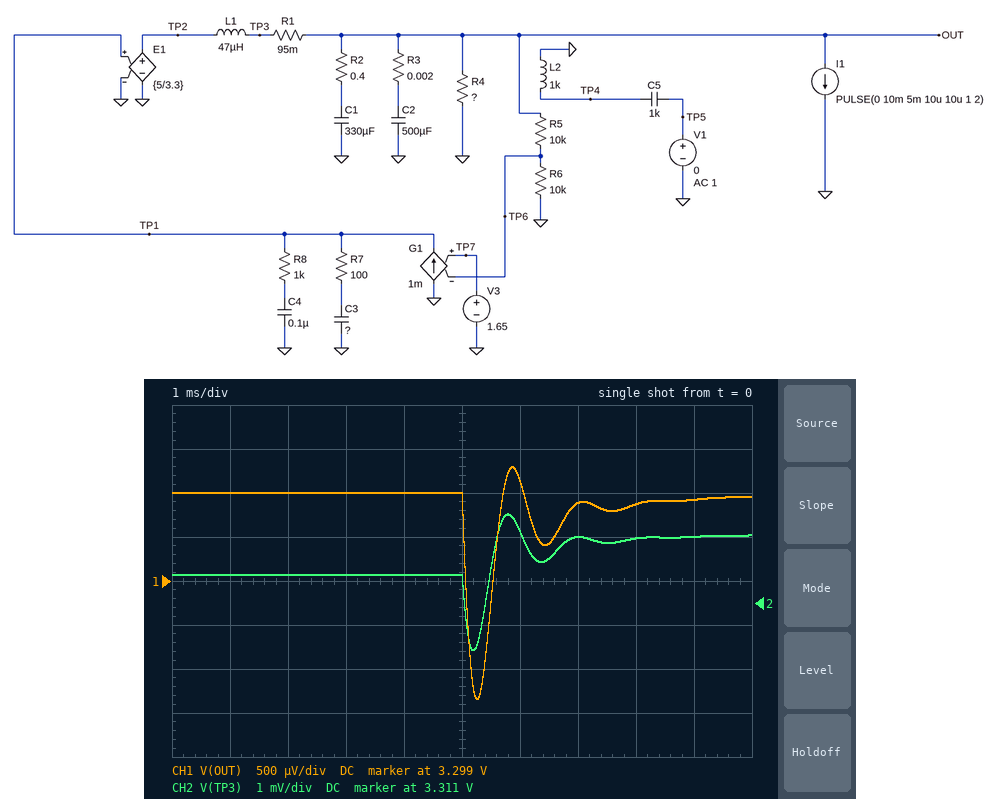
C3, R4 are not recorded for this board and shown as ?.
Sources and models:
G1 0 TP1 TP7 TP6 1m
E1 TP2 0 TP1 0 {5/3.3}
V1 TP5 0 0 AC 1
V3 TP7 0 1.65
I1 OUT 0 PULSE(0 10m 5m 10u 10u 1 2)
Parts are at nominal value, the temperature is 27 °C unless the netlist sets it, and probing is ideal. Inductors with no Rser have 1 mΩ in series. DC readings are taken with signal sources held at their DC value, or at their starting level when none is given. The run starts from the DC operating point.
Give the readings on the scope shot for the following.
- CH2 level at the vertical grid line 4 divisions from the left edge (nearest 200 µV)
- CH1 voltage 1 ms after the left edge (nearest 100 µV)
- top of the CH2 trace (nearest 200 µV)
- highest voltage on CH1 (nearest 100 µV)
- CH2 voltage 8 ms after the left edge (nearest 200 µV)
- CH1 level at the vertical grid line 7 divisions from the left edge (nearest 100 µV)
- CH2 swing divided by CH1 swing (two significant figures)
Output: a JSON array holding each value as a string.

["3.3116 V", "3.3000 V", "3.3130 V", "3.3003 V", "3.3124 V", "3.2999 V", "1.2"]
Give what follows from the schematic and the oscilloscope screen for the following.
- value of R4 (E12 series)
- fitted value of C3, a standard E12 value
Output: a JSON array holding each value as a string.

["27 Ω", "1.2 µF"]
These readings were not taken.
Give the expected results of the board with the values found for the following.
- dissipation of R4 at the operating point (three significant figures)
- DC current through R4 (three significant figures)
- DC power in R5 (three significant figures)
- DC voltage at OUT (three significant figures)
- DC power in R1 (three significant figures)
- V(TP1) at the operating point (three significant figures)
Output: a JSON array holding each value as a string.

["403 mW", "122 mA", "272 µW", "3.30 V", "1.42 mW", "2.19 V"]
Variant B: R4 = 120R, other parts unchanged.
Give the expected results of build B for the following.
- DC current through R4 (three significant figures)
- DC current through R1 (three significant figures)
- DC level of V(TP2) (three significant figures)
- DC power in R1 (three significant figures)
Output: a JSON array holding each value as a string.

["27.5 mA", "27.7 mA", "3.30 V", "72.7 µW"]
